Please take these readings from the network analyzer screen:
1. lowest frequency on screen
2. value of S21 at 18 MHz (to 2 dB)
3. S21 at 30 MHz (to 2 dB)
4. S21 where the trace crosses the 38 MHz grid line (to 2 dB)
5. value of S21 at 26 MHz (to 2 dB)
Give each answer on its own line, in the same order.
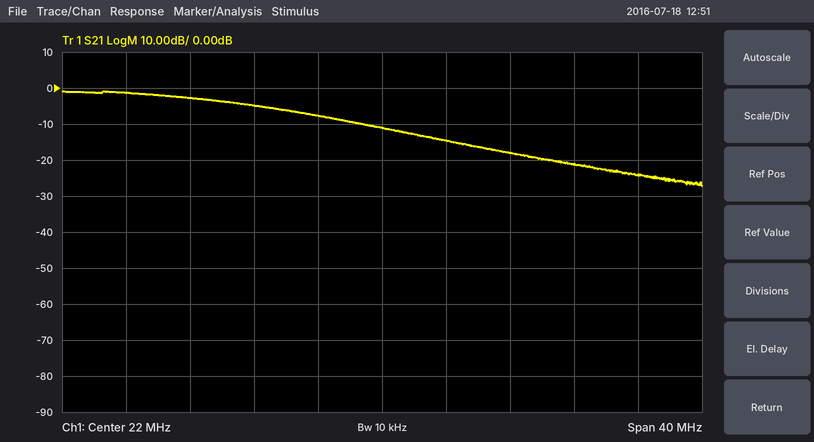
2 MHz
-8 dB
-18 dB
-24 dB
-14 dB
